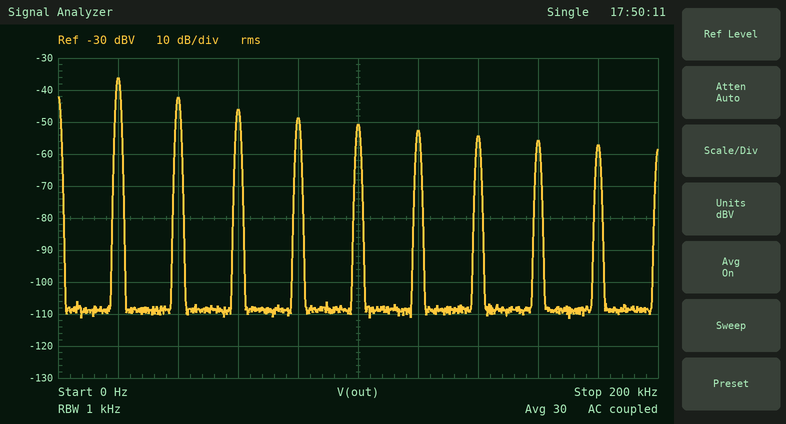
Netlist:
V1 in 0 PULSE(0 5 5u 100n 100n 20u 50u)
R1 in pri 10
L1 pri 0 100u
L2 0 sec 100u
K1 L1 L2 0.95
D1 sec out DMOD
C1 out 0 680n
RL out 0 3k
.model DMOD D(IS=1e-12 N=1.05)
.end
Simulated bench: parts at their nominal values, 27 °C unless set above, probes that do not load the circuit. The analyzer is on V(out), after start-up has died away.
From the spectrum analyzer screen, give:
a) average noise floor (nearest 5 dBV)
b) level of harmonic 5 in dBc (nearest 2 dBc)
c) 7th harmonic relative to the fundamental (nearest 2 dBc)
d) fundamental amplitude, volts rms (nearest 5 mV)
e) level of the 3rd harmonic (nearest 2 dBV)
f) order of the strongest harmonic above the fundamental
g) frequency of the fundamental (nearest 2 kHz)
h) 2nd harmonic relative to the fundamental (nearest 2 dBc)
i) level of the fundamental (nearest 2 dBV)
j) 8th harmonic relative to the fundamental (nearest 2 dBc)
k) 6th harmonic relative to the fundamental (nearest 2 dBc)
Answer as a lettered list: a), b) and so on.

a) -110 dBV
b) -14 dBc
c) -18 dBc
d) 15 mV
e) -46 dBV
f) 2
g) 20 kHz
h) -6 dBc
i) -36 dBV
j) -20 dBc
k) -16 dBc
